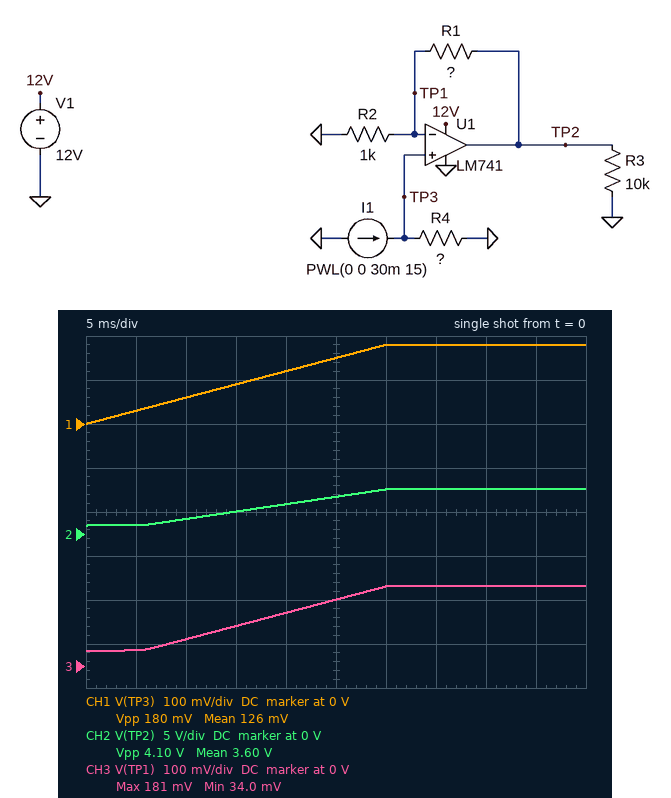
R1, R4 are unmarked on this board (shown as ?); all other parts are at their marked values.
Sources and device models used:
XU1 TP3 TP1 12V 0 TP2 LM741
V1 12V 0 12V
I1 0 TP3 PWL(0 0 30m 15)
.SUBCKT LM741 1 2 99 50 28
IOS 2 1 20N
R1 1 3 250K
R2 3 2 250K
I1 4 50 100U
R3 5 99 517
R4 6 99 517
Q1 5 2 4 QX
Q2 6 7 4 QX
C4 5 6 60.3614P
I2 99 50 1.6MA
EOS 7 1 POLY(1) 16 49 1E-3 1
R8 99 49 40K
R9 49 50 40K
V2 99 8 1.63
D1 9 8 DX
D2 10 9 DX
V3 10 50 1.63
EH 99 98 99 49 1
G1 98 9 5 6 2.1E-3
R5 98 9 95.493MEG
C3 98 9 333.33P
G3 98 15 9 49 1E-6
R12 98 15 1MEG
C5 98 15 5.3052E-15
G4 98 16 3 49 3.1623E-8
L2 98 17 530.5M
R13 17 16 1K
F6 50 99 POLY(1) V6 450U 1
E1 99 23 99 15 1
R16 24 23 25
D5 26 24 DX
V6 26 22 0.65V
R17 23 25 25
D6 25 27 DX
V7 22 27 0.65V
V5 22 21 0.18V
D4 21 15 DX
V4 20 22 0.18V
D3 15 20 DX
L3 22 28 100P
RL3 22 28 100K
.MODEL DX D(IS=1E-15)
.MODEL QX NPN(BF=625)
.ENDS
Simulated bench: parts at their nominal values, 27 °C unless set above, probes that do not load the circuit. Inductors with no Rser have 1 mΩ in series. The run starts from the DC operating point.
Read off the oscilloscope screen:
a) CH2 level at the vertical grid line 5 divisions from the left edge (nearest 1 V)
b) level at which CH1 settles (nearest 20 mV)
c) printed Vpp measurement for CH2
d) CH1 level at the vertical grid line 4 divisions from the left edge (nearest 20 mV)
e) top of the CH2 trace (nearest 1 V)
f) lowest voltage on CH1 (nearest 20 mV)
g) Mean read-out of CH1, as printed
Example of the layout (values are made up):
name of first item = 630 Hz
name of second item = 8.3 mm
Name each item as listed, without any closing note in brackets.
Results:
CH2 level at the vertical grid line 5 divisions from the left edge = 4 V
level at which CH1 settles = 180 mV
printed Vpp measurement for CH2 = 4.10 V
CH1 level at the vertical grid line 4 divisions from the left edge = 120 mV
top of the CH2 trace = 5 V
lowest voltage on CH1 = 0 V
Mean read-out of CH1, as printed = 126 mV
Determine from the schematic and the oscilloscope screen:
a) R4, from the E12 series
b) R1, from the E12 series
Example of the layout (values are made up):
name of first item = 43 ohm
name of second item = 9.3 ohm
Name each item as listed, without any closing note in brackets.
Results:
R4, from the E12 series = 0.012 Ω
R1, from the E12 series = 27 kΩ
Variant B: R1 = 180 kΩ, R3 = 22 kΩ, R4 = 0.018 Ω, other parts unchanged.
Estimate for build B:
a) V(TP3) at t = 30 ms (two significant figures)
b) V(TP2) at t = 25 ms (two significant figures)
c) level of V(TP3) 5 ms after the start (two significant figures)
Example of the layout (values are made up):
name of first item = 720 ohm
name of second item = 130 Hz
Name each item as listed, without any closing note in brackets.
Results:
V(TP3) at t = 30 ms = 270 mV
V(TP2) at t = 25 ms = 11 V
level of V(TP3) 5 ms after the start = 45 mV
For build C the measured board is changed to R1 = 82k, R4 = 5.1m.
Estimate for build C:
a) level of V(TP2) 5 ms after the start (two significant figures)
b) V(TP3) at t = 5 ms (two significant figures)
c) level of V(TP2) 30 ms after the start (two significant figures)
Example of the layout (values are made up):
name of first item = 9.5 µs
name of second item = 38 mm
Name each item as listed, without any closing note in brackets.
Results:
level of V(TP2) 5 ms after the start = 1.1 V
V(TP3) at t = 5 ms = 13 mV
level of V(TP2) 30 ms after the start = 6.4 V
